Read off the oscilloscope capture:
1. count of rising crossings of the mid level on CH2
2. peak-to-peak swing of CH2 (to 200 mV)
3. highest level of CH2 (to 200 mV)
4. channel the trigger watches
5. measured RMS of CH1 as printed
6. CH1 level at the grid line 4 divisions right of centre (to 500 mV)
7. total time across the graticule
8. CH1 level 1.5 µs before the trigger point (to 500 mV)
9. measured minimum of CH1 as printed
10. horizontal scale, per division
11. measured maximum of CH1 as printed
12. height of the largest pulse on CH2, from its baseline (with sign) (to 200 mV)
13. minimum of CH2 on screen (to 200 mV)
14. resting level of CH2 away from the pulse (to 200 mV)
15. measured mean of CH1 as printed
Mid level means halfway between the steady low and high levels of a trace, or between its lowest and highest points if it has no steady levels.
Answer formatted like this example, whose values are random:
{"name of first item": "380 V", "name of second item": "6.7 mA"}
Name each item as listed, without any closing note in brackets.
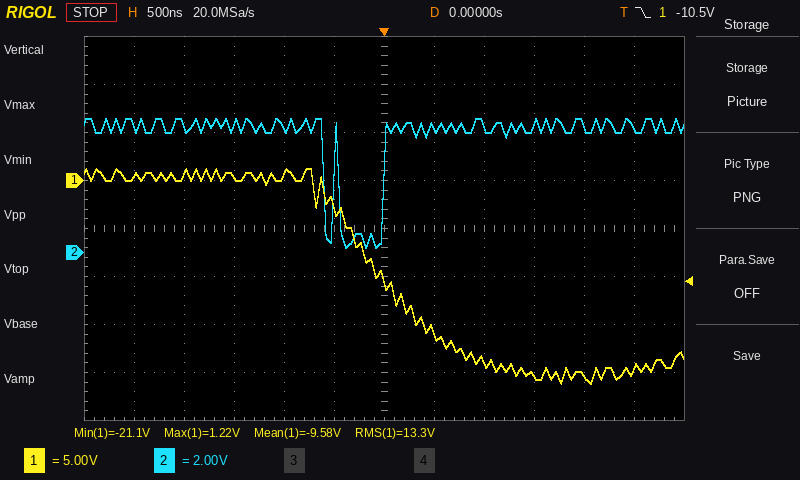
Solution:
{"count of rising crossings of the mid level on CH2": "2", "peak-to-peak swing of CH2": "5.4 V", "highest level of CH2": "5.6 V", "channel the trigger watches": "CH1", "measured RMS of CH1 as printed": "13.3 V", "CH1 level at the grid line 4 divisions right of centre": "-20.5 V", "total time across the graticule": "6 µs", "CH1 level 1.5 µs before the trigger point": "500 mV", "measured minimum of CH1 as printed": "-21.1 V", "horizontal scale, per division": "500 ns", "measured maximum of CH1 as printed": "1.22 V", "height of the largest pulse on CH2, from its baseline (with sign)": "-5.0 V", "minimum of CH2 on screen": "200 mV", "resting level of CH2 away from the pulse": "5.2 V", "measured mean of CH1 as printed": "-9.58 V"}
